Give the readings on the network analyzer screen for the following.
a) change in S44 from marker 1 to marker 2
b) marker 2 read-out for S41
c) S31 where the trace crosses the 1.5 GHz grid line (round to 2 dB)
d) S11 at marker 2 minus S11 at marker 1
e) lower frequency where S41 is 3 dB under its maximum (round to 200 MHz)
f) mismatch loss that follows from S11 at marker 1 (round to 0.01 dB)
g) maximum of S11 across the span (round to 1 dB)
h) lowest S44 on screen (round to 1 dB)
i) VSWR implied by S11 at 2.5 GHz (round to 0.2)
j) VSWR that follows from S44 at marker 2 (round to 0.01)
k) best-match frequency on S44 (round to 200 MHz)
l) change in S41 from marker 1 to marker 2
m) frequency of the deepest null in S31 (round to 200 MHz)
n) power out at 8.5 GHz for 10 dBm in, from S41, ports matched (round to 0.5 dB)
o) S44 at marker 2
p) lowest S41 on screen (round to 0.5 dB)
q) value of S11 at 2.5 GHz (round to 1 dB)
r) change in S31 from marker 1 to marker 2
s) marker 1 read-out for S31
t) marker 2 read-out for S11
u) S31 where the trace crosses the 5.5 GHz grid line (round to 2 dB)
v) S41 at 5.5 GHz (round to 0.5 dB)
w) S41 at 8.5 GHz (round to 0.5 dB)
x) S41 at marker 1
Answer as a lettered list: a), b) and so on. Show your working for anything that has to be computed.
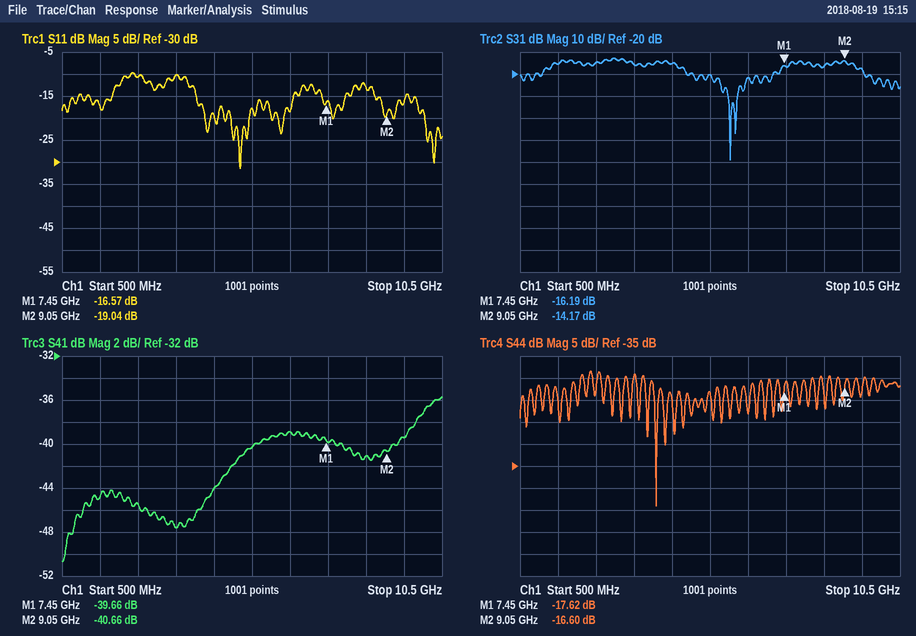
a) -16.6 − (-17.62) = 1.02 dB
b) -40.66 dB
c) -16 dB
d) -19.04 − (-16.57) = -2.47 dB
e) 9.6 GHz
f) −10 log10(1 − 10^(-16.57/10)) ≈ 0.10 dB
g) -10 dB
h) -44 dB
i) |Γ| = 10^(-11/20) = 0.2818; VSWR = (1 + 0.2818)/(1 − 0.2818) ≈ 1.8
j) (1 + 0.1479)/(1 − 0.1479) ≈ 1.35
k) 4.0 GHz
l) -40.66 − (-39.66) = -1.00 dB
m) 6.0 GHz
n) 10 dBm + (-41.0 dB) = -31.0 dBm
o) -16.60 dB
p) -50.5 dB
q) -11 dB
r) -14.17 − (-16.19) = 2.02 dB
s) -16.19 dB
t) -19.04 dB
u) -20 dB
v) -40.5 dB
w) -41.0 dB
x) -39.66 dB
